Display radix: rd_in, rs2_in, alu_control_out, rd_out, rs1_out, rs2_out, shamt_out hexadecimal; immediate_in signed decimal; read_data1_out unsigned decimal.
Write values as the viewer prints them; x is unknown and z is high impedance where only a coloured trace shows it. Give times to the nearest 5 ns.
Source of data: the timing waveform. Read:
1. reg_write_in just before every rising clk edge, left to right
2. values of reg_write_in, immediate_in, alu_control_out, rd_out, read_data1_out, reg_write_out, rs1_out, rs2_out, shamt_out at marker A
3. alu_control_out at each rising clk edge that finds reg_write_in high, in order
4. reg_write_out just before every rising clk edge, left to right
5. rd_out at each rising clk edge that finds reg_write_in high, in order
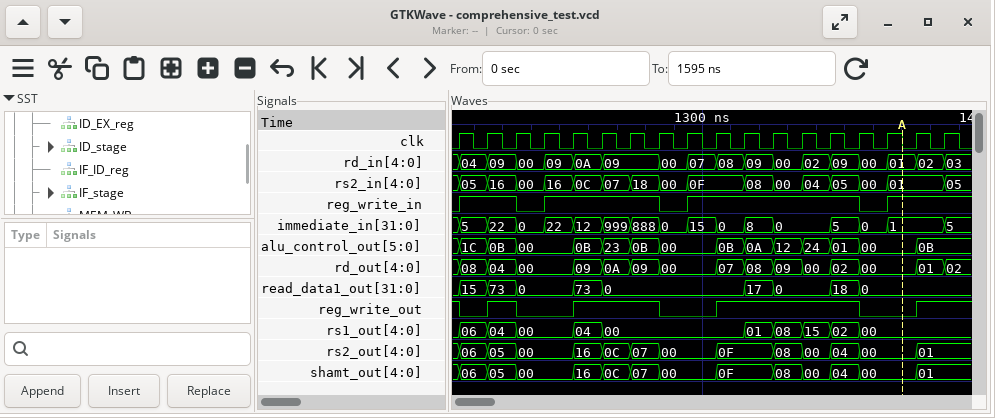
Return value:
0 1 1 0 1 1 1 1 0 1 1 1 1 1 1 0 1 1
reg_write_in=1, immediate_in=1, alu_control_out=00, rd_out=00, read_data1_out=0, reg_write_out=0, rs1_out=00, rs2_out=00, shamt_out=00
1C, 0B, 00, 0B, 23, 0B, 00, 0B, 0A, 12, 24, 01, 00, 0B
1 0 1 0 0 1 1 1 0 0 1 1 1 1 1 0 0 1
08, 04, 00, 09, 0A, 09, 00, 07, 08, 09, 00, 02, 00, 01
